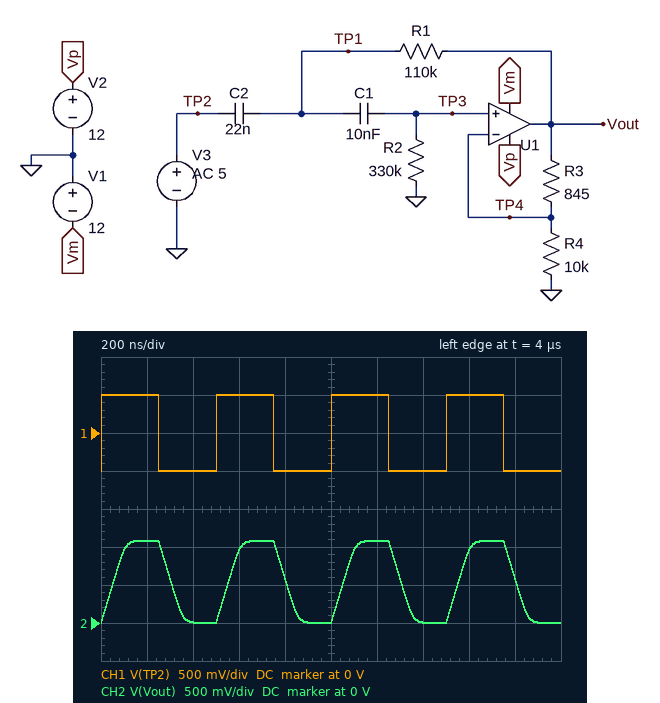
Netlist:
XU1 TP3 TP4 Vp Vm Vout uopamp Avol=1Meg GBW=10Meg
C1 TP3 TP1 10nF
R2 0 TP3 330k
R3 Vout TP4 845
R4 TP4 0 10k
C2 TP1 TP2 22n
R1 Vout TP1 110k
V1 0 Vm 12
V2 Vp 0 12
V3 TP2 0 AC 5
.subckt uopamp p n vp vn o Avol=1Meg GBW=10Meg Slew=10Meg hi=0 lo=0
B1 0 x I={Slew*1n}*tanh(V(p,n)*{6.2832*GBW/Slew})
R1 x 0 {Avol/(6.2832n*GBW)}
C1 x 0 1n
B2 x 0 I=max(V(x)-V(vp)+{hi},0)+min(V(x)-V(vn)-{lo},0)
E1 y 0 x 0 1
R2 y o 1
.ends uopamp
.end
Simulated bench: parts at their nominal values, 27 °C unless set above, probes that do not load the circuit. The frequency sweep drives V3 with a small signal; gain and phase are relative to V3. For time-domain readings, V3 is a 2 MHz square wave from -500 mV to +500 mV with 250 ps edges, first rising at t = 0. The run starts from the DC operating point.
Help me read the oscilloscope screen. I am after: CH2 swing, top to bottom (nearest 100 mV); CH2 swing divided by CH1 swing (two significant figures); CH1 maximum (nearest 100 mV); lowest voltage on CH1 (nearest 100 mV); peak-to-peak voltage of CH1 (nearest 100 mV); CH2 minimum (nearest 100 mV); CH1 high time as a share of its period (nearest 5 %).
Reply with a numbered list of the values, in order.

1. 1.1 V
2. 1.1
3. 500 mV
4. -500 mV
5. 1.0 V
6. 0 V
7. 50 %
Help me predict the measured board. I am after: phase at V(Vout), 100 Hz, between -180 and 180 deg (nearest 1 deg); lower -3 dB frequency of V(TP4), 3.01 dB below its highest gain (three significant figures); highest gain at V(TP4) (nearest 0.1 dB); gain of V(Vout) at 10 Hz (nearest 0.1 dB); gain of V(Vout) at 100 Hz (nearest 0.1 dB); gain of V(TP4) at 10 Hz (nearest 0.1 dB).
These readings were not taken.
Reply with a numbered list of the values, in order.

1. 43 deg
2. 49.7 Hz
3. 0.5 dB
4. -29.2 dB
5. 1.2 dB
6. -29.9 dB
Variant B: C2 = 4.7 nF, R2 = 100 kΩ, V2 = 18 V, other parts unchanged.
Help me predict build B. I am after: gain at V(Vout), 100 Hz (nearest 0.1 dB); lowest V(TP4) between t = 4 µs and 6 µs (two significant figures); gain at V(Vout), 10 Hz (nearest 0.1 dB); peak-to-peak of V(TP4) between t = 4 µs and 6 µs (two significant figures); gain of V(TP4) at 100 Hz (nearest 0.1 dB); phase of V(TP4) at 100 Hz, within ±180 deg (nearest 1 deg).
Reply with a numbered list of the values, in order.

1. -15.0 dB
2. -8.8 mV
3. -53.1 dB
4. 1.0 V
5. -15.7 dB
6. 130 deg
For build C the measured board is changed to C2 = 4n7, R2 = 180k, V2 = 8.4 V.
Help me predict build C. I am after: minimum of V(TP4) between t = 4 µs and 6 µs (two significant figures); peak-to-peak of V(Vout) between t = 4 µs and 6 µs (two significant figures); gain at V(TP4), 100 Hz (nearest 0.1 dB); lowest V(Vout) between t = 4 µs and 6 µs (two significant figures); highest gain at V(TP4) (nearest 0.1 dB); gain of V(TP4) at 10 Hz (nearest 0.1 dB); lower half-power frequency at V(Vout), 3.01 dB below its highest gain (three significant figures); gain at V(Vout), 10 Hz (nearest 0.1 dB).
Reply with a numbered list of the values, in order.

1. -4.7 mV
2. 1.1 V
3. -9.7 dB
4. -5.1 mV
5. 0 dB
6. -48.7 dB
7. 178 Hz
8. -48.0 dB
